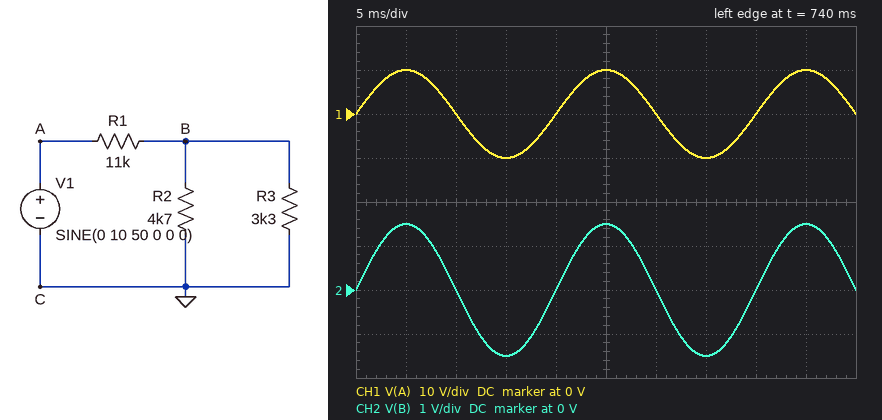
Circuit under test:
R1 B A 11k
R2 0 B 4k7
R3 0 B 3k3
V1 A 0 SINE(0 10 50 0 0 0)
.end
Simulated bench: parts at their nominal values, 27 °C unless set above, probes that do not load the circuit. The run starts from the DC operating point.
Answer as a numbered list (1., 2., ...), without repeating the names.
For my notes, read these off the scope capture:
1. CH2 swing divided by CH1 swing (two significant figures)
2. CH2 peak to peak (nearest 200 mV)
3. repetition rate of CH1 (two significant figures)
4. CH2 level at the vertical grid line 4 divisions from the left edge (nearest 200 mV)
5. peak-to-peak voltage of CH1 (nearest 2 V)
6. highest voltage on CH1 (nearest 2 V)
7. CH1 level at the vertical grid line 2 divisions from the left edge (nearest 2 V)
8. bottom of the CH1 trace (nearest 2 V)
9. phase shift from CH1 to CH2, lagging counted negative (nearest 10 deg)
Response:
1. 0.15
2. 3.0 V
3. 50 Hz
4. 0 V
5. 20 V
6. 10 V
7. 0 V
8. -10 V
9. 0 deg
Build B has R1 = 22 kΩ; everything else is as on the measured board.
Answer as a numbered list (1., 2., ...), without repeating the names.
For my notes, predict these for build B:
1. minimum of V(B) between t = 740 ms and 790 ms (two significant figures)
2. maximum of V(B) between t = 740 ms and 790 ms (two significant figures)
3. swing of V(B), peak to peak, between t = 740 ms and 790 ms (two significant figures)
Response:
1. -810 mV
2. 810 mV
3. 1.6 V
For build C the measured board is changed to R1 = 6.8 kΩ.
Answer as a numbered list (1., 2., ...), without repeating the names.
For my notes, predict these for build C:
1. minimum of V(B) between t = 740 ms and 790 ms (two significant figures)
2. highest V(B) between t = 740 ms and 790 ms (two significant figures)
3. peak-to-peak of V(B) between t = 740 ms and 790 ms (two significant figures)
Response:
1. -2.2 V
2. 2.2 V
3. 4.4 V
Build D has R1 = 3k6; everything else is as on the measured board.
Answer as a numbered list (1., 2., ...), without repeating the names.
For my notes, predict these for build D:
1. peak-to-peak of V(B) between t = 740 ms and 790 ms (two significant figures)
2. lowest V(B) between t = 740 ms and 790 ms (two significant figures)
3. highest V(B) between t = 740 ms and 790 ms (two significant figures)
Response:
1. 7.0 V
2. -3.5 V
3. 3.5 V
